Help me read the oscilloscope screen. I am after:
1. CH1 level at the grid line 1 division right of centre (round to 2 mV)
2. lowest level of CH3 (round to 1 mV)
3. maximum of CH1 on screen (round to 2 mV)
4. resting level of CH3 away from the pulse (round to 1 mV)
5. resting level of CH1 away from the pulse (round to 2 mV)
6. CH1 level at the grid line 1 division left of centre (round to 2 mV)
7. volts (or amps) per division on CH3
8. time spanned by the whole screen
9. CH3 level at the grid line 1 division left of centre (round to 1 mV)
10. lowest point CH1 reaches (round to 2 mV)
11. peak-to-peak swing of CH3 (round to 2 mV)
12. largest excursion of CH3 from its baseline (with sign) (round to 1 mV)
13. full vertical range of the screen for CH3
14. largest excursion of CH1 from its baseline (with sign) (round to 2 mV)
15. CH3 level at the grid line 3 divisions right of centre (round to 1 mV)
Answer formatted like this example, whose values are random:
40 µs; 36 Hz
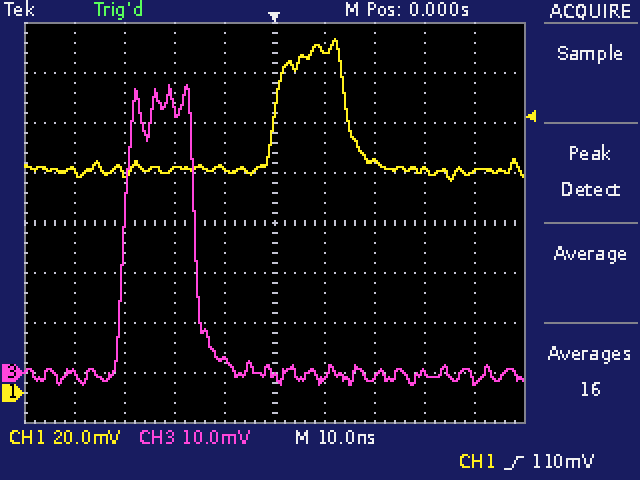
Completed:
138 mV; -2 mV; 142 mV; 0 mV; 90 mV; 90 mV; 10 mV; 100 ns; 3 mV; 84 mV; 60 mV; +58 mV; 80 mV; +52 mV; 0 mV
